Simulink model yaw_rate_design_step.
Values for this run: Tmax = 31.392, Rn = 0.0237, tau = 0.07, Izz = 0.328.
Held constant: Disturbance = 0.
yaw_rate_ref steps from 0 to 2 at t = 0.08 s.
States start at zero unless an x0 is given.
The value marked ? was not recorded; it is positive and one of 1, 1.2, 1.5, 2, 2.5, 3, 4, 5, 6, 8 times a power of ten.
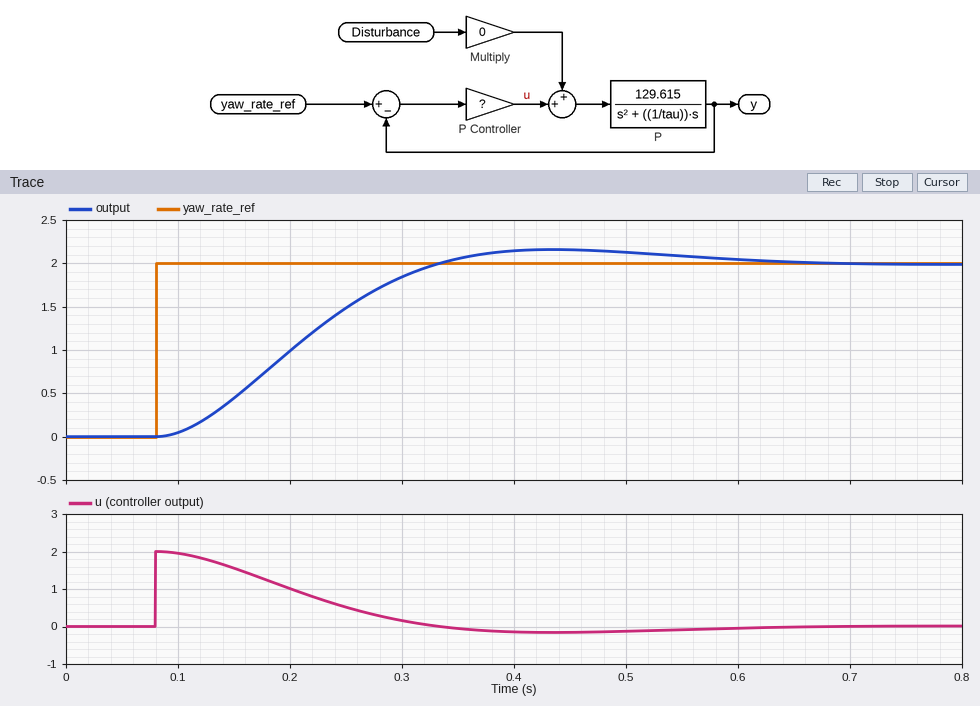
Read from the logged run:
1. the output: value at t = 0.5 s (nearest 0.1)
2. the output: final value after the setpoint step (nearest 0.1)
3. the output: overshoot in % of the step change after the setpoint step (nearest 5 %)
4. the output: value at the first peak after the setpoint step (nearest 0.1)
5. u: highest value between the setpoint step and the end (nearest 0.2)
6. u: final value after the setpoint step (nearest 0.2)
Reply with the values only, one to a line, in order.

2.1
2.0
10 %
2.2
2.0
0.0
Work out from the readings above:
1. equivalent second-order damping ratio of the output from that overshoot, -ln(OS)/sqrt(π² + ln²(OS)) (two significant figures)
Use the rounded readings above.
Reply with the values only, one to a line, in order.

0.59
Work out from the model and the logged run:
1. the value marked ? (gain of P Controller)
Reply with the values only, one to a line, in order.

1
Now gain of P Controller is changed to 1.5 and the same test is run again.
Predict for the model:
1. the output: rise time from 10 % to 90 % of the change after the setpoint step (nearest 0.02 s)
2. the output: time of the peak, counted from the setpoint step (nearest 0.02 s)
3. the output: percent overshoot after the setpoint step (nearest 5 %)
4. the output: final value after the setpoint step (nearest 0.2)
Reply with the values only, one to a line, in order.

0.12 s
0.26 s
15 %
2.0
